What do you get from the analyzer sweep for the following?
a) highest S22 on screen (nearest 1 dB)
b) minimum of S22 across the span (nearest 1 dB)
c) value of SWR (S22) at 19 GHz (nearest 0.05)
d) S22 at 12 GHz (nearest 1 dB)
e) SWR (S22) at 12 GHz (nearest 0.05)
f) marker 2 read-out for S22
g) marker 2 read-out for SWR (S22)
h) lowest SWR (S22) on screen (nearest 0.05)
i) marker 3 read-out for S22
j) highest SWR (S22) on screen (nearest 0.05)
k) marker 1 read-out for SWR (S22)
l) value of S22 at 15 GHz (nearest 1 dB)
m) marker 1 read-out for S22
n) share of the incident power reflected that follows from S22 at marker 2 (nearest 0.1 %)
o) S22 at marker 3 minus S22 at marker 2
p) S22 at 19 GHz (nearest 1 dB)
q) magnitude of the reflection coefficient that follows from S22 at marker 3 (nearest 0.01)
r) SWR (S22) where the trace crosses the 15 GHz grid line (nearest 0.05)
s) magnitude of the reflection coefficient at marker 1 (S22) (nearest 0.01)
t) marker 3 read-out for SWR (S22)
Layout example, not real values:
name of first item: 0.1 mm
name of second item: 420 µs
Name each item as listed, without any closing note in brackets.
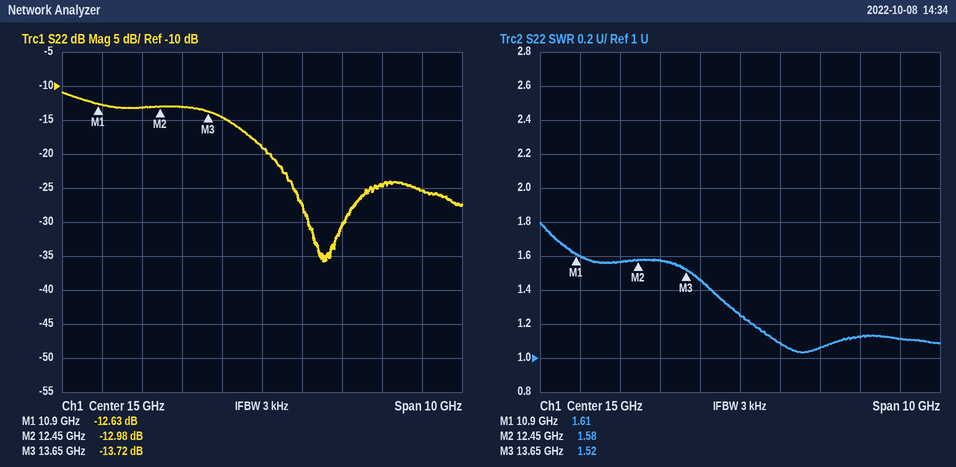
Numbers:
highest S22 on screen: -11 dB
minimum of S22 across the span: -36 dB
value of SWR (S22) at 19 GHz: 1.10
S22 at 12 GHz: -13 dB
SWR (S22) at 12 GHz: 1.55
marker 2 read-out for S22: -12.98 dB
marker 2 read-out for SWR: 1.58
lowest SWR (S22) on screen: 1.05
marker 3 read-out for S22: -13.72 dB
highest SWR (S22) on screen: 1.80
marker 1 read-out for SWR: 1.61
value of S22 at 15 GHz: -19 dB
marker 1 read-out for S22: -12.63 dB
share of the incident power reflected that follows from S22 at marker 2: 5.0 %
S22 at marker 3 minus S22 at marker 2: -0.74 dB
S22 at 19 GHz: -25 dB
magnitude of the reflection coefficient that follows from S22 at marker 3: 0.21
SWR (S22) where the trace crosses the 15 GHz grid line: 1.25
magnitude of the reflection coefficient at marker 1 (S22): 0.23
marker 3 read-out for SWR: 1.52
